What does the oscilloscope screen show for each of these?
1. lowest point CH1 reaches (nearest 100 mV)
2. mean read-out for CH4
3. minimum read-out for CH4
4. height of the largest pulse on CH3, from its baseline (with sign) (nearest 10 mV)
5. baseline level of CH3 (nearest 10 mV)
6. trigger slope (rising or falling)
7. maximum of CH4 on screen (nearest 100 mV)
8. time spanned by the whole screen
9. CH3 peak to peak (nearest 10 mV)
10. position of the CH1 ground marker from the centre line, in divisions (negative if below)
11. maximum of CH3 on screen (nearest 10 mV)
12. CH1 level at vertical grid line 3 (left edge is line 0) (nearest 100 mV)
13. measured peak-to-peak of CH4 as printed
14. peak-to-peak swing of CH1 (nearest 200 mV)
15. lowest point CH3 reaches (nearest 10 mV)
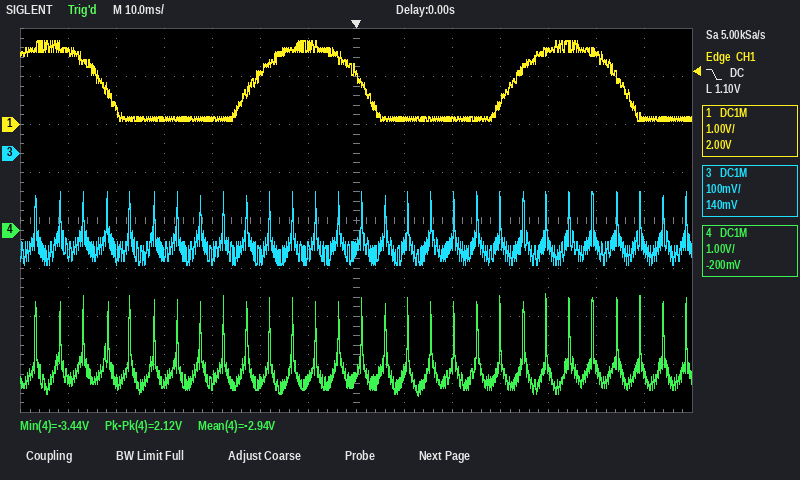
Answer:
100 mV
-2.94 V
-3.44 V
+120 mV
-200 mV
falling
-1.3 V
140 ms
150 mV
+2.0 div
-80 mV
100 mV
2.12 V
1.6 V
-230 mV
